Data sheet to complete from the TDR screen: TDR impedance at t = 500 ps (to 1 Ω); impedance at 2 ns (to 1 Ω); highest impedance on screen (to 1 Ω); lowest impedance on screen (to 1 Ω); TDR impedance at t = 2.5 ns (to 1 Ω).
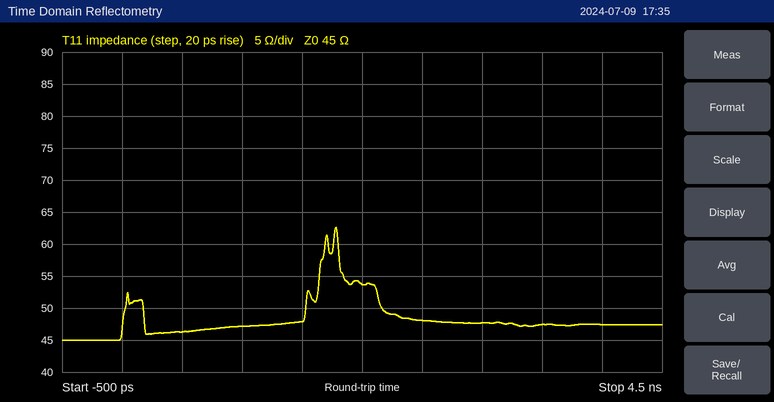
46 Ω
54 Ω
63 Ω
45 Ω
48 Ω
